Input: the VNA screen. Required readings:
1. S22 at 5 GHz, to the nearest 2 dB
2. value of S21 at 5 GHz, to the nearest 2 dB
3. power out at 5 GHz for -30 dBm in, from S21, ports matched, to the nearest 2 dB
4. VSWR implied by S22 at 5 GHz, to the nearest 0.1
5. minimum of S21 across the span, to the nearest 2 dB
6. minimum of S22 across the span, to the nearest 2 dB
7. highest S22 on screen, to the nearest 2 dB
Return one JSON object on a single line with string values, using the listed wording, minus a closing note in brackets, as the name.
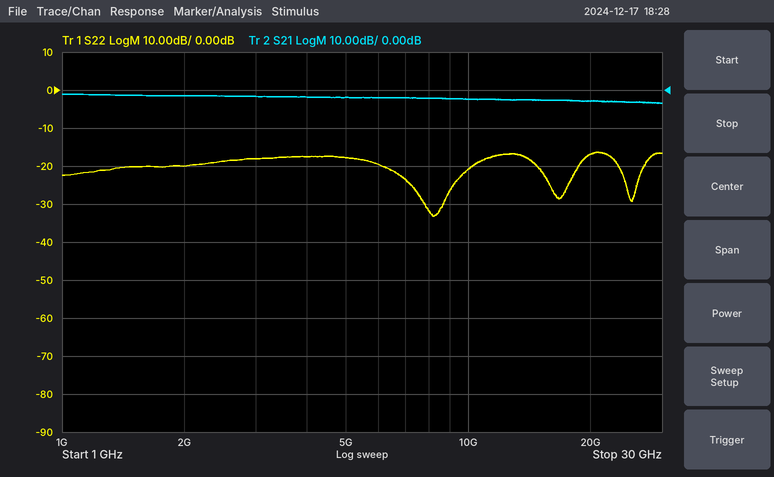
{"S22 at 5 GHz, to the nearest 2 dB": "-18 dB", "value of S21 at 5 GHz, to the nearest 2 dB": "-2 dB", "power out at 5 GHz for -30 dBm in, from S21, ports matched, to the nearest 2 dB": "-32 dBm", "VSWR implied by S22 at 5 GHz, to the nearest 0.1": "1.3", "minimum of S21 across the span, to the nearest 2 dB": "-4 dB", "minimum of S22 across the span, to the nearest 2 dB": "-34 dB", "highest S22 on screen, to the nearest 2 dB": "-16 dB"}
